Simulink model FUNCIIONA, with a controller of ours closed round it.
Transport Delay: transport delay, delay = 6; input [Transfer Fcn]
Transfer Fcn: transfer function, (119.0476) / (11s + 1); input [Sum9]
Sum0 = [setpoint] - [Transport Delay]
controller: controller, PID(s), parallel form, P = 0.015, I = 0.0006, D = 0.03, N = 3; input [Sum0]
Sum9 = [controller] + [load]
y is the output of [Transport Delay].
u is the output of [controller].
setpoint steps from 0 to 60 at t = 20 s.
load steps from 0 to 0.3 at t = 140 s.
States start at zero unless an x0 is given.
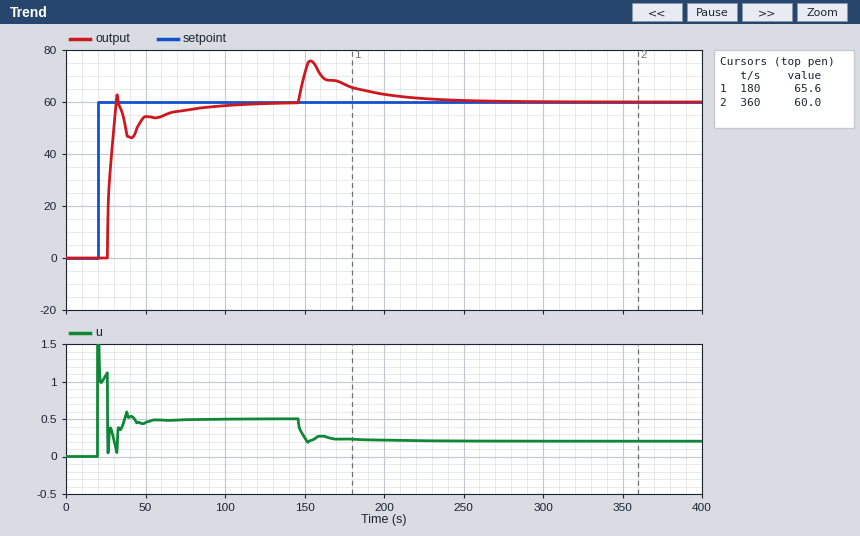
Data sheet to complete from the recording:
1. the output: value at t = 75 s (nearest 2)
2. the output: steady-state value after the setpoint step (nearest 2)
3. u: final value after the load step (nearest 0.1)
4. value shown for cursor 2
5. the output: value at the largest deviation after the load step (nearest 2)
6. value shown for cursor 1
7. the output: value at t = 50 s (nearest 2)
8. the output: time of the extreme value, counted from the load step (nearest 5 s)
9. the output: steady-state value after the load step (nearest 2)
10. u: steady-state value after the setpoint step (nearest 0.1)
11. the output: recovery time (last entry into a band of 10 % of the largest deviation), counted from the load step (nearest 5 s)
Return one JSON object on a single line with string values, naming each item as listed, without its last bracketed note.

{"the output: value at t = 75 s": "56", "the output: steady-state value after the setpoint step": "60", "u: final value after the load step": "0.2", "value shown for cursor 2": "60.0", "the output: value at the largest deviation after the load step": "76", "value shown for cursor 1": "65.6", "the output: value at t = 50 s": "54", "the output: time of the extreme value, counted from the load step": "15 s", "the output: steady-state value after the load step": "60", "u: steady-state value after the setpoint step": "0.5", "the output: recovery time (last entry into a band of 10 % of the largest deviation), counted from the load step": "80 s"}
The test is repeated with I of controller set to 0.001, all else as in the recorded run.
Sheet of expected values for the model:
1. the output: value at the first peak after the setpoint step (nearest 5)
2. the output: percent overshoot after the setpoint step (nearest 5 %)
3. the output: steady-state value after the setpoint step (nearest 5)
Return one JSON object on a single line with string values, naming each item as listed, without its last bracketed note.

{"the output: value at the first peak after the setpoint step": "65", "the output: percent overshoot after the setpoint step": "10 %", "the output: steady-state value after the setpoint step": "60"}
